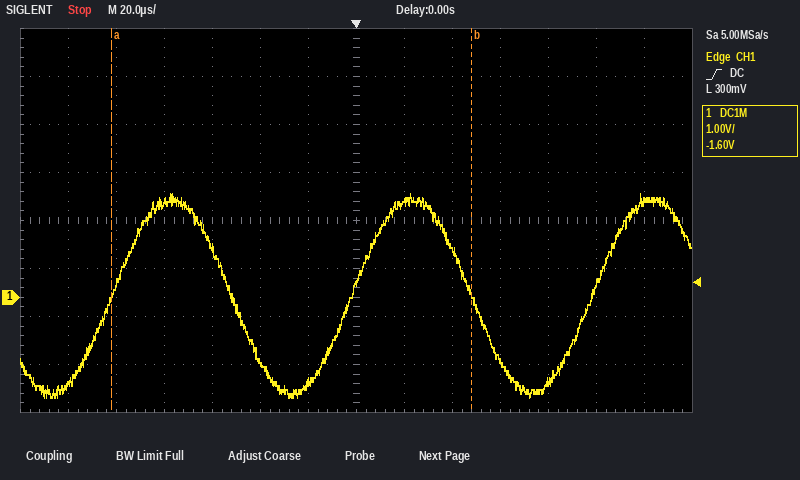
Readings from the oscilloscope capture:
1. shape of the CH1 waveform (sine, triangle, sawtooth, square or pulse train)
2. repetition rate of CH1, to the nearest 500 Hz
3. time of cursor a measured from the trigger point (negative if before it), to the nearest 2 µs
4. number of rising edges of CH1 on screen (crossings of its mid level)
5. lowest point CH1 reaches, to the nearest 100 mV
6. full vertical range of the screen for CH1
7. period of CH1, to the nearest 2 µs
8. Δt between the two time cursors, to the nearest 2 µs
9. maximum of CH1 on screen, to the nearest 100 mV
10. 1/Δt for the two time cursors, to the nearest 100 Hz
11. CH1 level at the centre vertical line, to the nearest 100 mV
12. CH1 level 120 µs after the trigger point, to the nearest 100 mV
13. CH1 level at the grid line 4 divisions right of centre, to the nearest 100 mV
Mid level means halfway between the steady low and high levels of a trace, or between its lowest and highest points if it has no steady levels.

sine
10.0 kHz
-102 µs
3
-2.1 V
8 V
100 µs
150 µs
2.2 V
6.7 kHz
300 mV
2.0 V
-1.8 V
